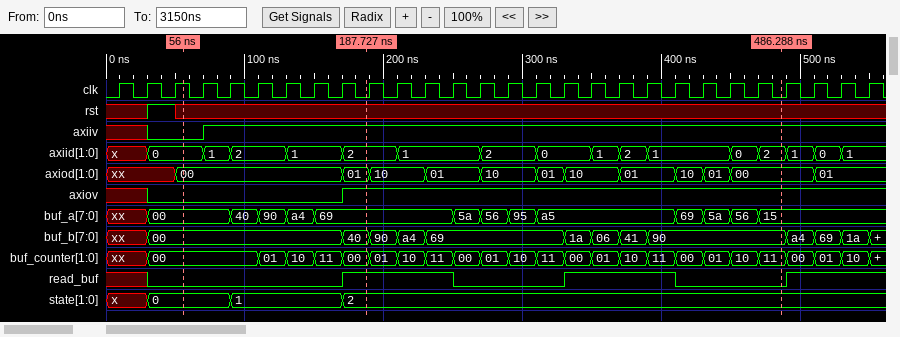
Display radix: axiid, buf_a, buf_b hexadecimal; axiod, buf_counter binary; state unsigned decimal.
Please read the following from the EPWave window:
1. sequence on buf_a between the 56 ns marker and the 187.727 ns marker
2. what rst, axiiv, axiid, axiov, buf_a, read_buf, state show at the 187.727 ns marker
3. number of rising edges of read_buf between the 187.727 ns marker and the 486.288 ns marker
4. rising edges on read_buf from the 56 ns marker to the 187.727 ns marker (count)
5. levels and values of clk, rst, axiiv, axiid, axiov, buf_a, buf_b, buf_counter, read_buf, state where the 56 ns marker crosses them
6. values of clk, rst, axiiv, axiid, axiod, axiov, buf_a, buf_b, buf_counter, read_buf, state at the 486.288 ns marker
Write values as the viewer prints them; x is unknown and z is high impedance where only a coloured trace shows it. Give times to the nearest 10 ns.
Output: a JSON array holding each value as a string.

["00, 40, 90, a4, 69", "rst=x, axiiv=1, axiid=2, axiov=1, buf_a=69, read_buf=1, state=2", "1", "1", "clk=1, rst=x, axiiv=0, axiid=0, axiov=0, buf_a=00, buf_b=00, buf_counter=00, read_buf=0, state=0", "clk=0, rst=x, axiiv=1, axiid=2, axiod=00, axiov=1, buf_a=15, buf_b=90, buf_counter=11, read_buf=0, state=2"]
